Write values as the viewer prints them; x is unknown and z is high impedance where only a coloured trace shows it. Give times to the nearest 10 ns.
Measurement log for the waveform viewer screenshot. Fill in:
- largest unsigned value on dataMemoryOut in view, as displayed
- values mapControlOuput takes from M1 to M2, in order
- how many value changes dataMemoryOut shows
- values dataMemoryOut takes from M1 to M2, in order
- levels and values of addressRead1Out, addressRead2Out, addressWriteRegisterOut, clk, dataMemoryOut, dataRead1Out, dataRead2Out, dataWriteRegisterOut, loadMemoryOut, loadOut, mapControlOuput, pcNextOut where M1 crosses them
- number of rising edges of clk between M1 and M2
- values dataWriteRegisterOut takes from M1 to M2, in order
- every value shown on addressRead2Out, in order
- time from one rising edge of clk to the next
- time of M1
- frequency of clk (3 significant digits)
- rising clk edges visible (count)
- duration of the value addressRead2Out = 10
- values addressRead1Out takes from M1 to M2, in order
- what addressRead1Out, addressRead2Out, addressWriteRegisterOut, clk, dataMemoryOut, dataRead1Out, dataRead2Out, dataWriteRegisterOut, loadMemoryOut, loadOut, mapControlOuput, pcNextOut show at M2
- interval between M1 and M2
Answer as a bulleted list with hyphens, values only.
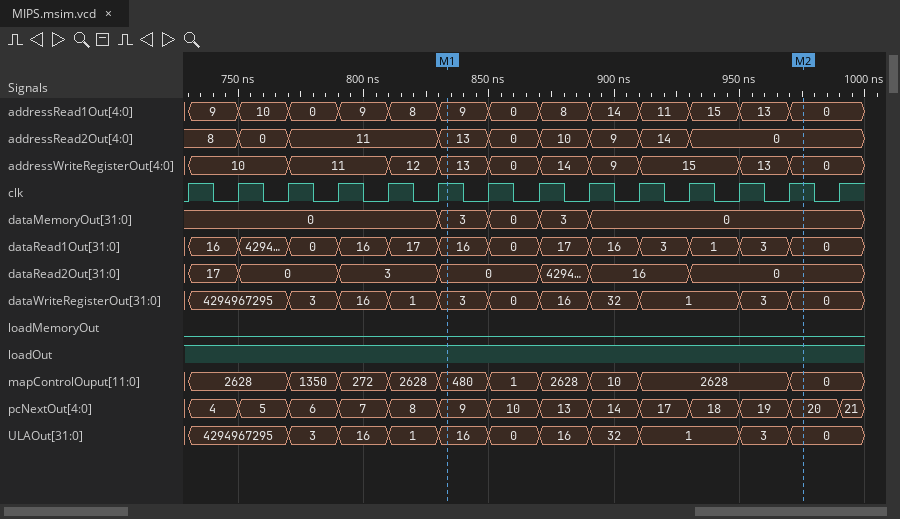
- 3
- 480, 1, 2628, 10, 2628, 0
- 4
- 3, 0, 3, 0
- addressRead1Out=9, addressRead2Out=13, addressWriteRegisterOut=13, clk=1, dataMemoryOut=3, dataRead1Out=16, dataRead2Out=0, dataWriteRegisterOut=3, loadMemoryOut=0, loadOut=1, mapControlOuput=480, pcNextOut=9
- 7
- 3, 0, 16, 32, 1, 3, 0
- 8, 0, 11, 13, 0, 10, 9, 14, 0
- 20 ns
- 830 ns
- 50.0 MHz
- 14
- 20 ns
- 9, 0, 8, 14, 11, 15, 13, 0
- addressRead1Out=0, addressRead2Out=0, addressWriteRegisterOut=0, clk=1, dataMemoryOut=0, dataRead1Out=0, dataRead2Out=0, dataWriteRegisterOut=0, loadMemoryOut=0, loadOut=1, mapControlOuput=0, pcNextOut=20
- 140 ns
